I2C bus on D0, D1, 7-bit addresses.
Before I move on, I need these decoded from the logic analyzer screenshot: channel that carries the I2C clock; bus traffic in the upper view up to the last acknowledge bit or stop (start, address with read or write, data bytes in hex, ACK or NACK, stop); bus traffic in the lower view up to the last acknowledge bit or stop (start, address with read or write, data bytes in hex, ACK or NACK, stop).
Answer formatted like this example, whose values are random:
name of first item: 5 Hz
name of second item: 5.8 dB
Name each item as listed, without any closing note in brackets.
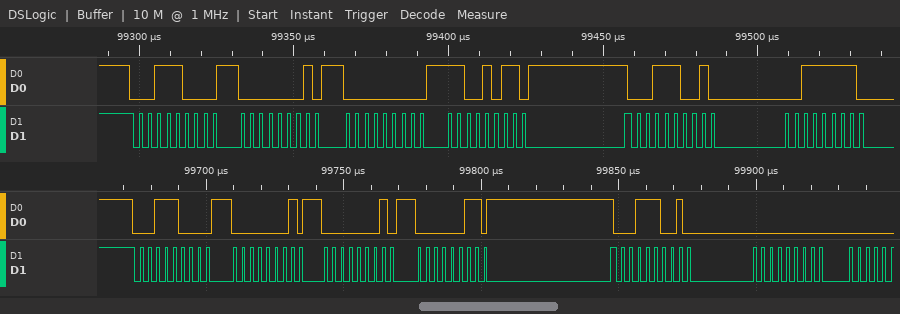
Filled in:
channel that carries the I2C clock: D1
bus traffic in the upper view up to the last acknowledge bit or stop: start, address 1C write ACK, 01 ACK, 00 ACK, CB ACK, repeated start, address 1C read ACK, 3F ACK
bus traffic in the lower view up to the last acknowledge bit or stop: start, address 1C write ACK, 01 ACK, 01 ACK, 03 ACK, repeated start, address 1C read ACK, 00 ACK
